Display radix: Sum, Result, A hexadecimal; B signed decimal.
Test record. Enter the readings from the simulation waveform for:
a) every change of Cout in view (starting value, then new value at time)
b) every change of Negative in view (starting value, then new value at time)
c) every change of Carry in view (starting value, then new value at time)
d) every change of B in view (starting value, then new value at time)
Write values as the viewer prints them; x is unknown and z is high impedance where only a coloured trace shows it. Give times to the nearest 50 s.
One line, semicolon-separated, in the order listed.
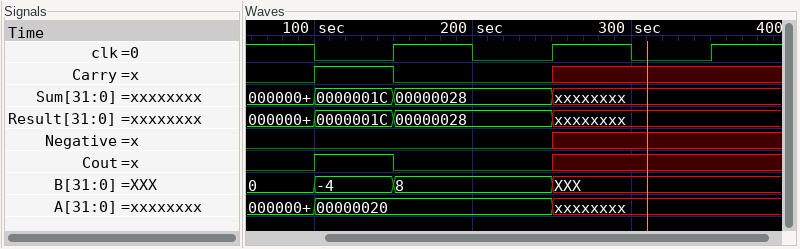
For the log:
0, 1 at 100 s, 0 at 150 s, x at 250 s; 0, x at 250 s; 0, 1 at 100 s, 0 at 150 s, x at 250 s; 0, -4 at 100 s, 8 at 150 s, XXX at 250 s
